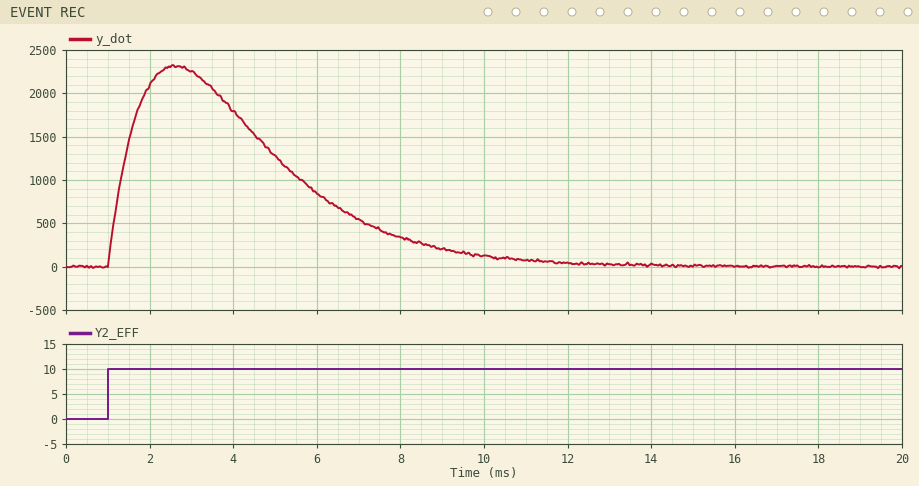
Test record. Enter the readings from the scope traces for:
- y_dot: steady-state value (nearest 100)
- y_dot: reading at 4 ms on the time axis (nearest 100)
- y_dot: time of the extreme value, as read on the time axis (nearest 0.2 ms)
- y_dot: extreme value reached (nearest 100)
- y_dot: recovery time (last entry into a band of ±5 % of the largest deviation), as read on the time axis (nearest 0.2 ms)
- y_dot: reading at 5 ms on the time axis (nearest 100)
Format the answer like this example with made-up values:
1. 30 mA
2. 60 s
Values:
1. 0
2. 1800
3. 2.6 ms
4. 2300
5. 10.2 ms
6. 1300
